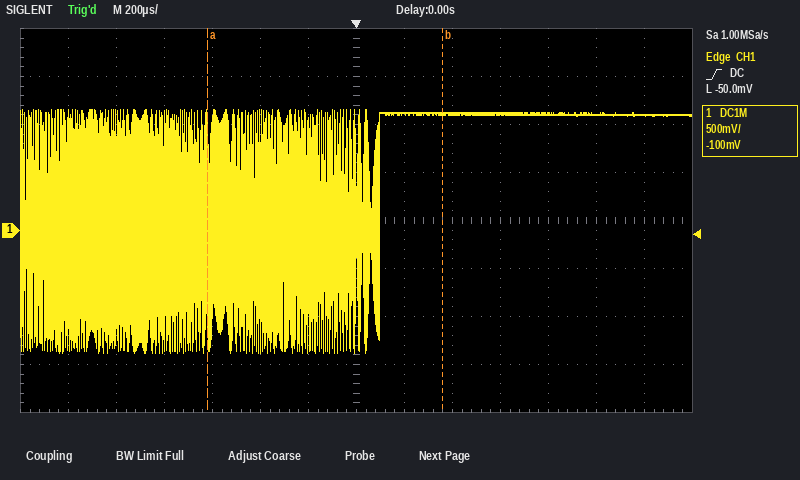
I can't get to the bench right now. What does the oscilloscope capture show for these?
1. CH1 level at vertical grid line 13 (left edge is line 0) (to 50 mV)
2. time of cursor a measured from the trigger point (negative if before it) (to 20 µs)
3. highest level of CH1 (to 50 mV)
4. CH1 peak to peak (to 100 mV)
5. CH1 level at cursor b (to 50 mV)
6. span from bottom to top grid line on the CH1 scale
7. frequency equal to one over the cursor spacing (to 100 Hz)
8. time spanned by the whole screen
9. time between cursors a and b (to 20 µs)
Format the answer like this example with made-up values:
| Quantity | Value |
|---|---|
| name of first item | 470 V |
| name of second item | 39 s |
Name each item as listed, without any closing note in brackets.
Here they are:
| Quantity | Value |
|---|---|
| CH1 level at vertical grid line 13 (left edge is line 0) | 1.20 V |
| time of cursor a measured from the trigger point (negative if before it) | -620 µs |
| highest level of CH1 | 1.25 V |
| CH1 peak to peak | 2.50 V |
| CH1 level at cursor b | 1.20 V |
| span from bottom to top grid line on the CH1 scale | 4 V |
| frequency equal to one over the cursor spacing | 1.0 kHz |
| time spanned by the whole screen | 2.8 ms |
| time between cursors a and b | 980 µs |
